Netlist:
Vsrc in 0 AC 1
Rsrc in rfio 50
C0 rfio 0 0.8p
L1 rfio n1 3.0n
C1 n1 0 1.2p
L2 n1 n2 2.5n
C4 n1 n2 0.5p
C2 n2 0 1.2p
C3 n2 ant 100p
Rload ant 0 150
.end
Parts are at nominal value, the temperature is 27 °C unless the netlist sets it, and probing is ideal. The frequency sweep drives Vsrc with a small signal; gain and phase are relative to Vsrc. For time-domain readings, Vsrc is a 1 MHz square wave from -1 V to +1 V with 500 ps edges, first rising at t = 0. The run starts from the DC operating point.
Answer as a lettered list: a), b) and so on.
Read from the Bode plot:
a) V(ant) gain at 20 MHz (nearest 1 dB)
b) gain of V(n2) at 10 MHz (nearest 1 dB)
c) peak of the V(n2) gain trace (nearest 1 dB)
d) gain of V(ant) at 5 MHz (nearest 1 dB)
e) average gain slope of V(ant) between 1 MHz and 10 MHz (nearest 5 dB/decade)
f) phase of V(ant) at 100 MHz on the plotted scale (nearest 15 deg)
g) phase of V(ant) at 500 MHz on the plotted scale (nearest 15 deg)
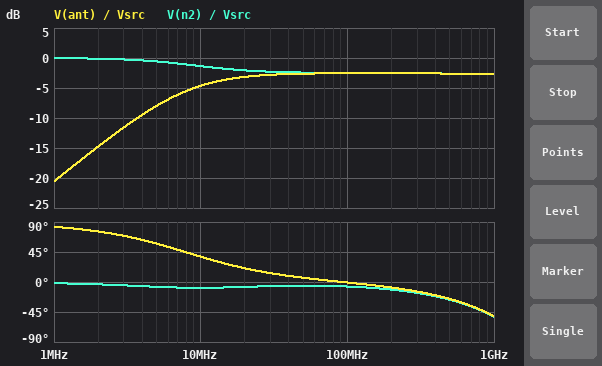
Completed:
a) -3 dB
b) -1 dB
c) 0 dB
d) -8 dB
e) 15 dB/decade
f) 0 deg
g) -30 deg
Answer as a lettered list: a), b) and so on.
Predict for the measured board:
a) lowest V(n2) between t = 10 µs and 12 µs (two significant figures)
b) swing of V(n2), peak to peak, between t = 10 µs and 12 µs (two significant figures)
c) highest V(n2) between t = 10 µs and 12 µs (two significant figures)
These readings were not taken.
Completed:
a) -1.0 V
b) 2.0 V
c) 1.0 V
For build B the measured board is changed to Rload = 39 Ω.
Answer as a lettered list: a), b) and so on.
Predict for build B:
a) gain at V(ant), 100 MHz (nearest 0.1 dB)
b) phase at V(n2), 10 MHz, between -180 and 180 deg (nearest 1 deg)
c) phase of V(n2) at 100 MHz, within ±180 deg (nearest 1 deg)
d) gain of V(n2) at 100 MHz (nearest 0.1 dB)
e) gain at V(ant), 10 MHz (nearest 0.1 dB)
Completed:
a) -7.3 dB
b) -16 deg
c) -17 deg
d) -6.7 dB
e) -13.4 dB
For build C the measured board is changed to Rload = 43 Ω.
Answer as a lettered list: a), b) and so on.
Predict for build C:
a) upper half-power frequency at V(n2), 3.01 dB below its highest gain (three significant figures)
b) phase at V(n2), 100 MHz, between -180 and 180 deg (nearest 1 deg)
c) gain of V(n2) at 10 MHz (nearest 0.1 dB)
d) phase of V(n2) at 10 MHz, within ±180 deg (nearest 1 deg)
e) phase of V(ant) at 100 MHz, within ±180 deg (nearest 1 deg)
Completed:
a) 22.5 MHz
b) -15 deg
c) -1.0 dB
d) -16 deg
e) 5 deg
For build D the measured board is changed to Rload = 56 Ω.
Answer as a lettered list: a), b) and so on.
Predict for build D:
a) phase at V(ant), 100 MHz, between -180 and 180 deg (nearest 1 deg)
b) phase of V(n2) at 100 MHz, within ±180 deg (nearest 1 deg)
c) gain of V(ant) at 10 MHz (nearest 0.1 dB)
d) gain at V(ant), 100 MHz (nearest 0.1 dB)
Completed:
a) 4 deg
b) -12 deg
c) -10.7 dB
d) -5.7 dB
